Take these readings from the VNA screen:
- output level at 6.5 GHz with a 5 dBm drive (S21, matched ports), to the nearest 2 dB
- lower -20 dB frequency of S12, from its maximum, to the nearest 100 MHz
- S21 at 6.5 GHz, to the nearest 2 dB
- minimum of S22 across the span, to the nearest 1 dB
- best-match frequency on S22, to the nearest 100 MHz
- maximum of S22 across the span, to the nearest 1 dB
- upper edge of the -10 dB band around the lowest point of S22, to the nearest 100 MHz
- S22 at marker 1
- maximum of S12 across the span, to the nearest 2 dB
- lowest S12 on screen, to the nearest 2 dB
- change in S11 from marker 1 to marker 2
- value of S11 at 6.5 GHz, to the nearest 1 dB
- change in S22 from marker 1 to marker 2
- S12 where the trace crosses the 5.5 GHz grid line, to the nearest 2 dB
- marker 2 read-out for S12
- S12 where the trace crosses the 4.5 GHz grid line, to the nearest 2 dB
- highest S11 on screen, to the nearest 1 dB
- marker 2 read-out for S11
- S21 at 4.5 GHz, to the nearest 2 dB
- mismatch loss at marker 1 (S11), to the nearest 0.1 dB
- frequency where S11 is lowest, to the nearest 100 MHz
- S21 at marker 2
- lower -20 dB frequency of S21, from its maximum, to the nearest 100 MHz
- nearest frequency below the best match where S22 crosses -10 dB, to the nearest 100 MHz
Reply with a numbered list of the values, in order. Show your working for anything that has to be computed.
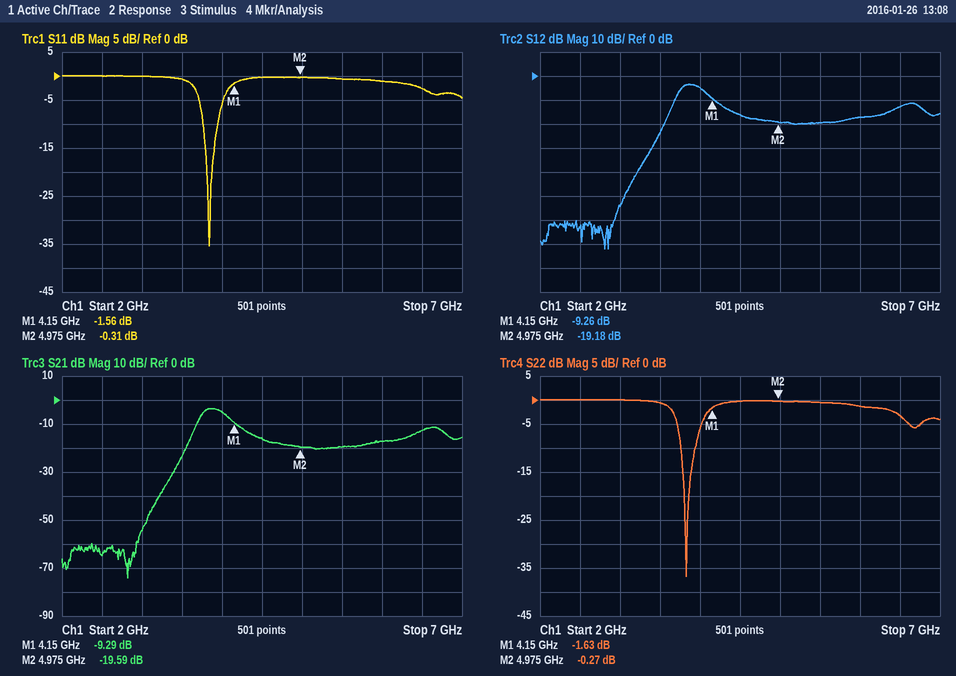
1. 5 dBm + (-12 dB) = -8 dBm
2. 3.5 GHz
3. -12 dB
4. -37 dB
5. 3.8 GHz
6. 0 dB
7. 3.9 GHz
8. -1.63 dB
9. -4 dB
10. -72 dB
11. -0.31 − (-1.56) = 1.25 dB
12. -3 dB
13. -0.27 − (-1.63) = 1.36 dB
14. -20 dB
15. -19.18 dB
16. -16 dB
17. 0 dB
18. -0.31 dB
19. -16 dB
20. −10 log10(1 − 10^(-1.56/10)) ≈ 5.2 dB
21. 3.8 GHz
22. -19.59 dB
23. 3.5 GHz
24. 3.8 GHz
